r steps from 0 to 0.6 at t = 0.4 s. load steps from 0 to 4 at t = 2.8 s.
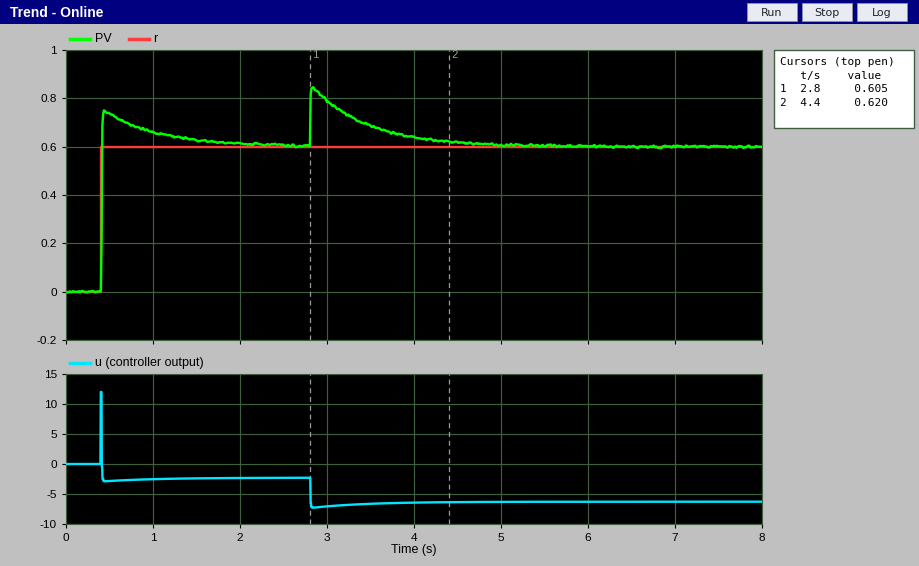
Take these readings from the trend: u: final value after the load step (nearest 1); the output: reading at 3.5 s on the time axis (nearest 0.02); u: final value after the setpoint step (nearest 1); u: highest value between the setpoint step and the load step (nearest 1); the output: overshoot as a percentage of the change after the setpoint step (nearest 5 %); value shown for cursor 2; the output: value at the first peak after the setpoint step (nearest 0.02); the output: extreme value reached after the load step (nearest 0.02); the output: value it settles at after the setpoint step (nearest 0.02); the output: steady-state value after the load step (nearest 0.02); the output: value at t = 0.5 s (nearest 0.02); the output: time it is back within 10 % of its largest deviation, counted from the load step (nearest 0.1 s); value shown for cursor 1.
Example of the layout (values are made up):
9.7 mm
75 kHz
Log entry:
-6
0.68
-2
12
25 %
0.620
0.74
0.84
0.60
0.60
0.74
1.5 s
0.605
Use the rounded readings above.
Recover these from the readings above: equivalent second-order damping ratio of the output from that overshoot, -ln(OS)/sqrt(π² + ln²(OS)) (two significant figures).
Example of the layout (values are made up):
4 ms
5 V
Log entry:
0.40
